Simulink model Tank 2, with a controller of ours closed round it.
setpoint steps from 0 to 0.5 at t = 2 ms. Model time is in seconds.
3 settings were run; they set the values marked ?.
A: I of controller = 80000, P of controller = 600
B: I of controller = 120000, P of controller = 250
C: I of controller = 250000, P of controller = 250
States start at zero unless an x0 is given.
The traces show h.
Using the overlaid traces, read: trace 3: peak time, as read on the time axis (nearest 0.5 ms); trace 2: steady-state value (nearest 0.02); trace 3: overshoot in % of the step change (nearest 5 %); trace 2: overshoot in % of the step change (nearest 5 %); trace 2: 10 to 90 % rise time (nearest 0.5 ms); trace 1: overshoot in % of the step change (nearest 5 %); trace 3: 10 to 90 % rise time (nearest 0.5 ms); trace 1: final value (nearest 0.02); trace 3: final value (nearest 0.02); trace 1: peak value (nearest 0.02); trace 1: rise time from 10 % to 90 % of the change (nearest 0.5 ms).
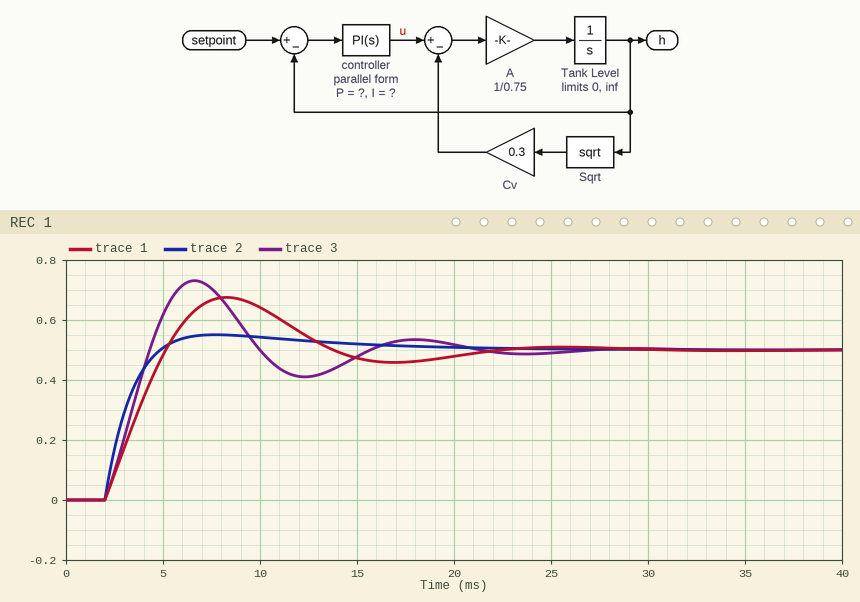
6.5 ms
0.50
45 %
10 %
2.0 ms
35 %
2.0 ms
0.50
0.50
0.68
2.5 ms
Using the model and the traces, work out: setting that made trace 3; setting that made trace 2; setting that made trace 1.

C
A
B
